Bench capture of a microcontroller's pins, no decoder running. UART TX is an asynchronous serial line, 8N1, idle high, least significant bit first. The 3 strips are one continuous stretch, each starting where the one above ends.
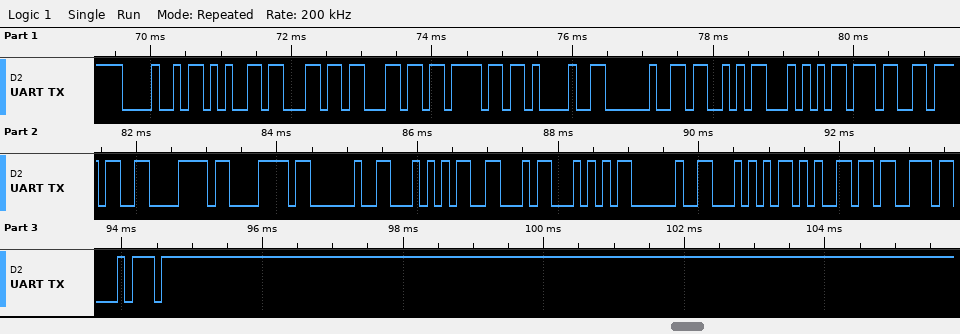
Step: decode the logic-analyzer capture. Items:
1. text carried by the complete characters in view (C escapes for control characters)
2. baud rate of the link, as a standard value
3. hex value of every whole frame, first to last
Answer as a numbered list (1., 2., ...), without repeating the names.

1. "Hello! ST77xx TFT Test"
2. 9600 baud
3. 0x48 0x65 0x6C 0x6C 0x6F 0x21 0x20 0x53 0x54 0x37 0x37 0x78 0x78 0x20 0x54 0x46 0x54 0x20 0x54 0x65 0x73 0x74
